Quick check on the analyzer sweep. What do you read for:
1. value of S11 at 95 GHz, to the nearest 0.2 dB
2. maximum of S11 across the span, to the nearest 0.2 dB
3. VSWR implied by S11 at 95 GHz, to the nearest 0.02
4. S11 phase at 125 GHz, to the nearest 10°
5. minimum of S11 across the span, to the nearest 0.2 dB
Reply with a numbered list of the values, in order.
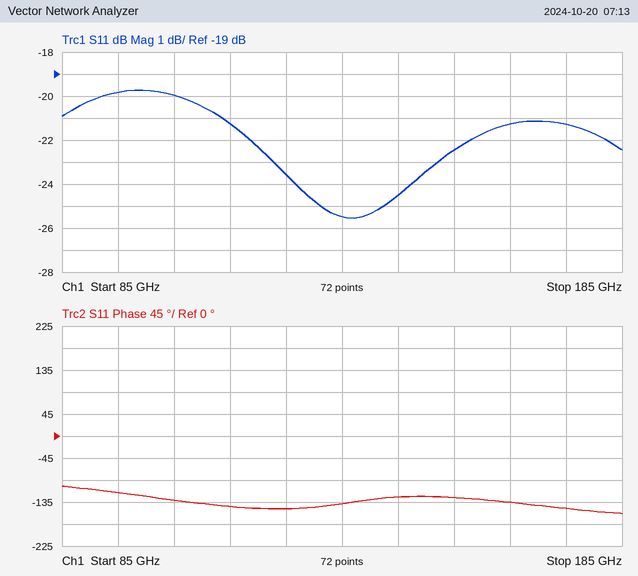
1. -19.8 dB
2. -19.8 dB
3. 1.22
4. -150°
5. -25.6 dB
